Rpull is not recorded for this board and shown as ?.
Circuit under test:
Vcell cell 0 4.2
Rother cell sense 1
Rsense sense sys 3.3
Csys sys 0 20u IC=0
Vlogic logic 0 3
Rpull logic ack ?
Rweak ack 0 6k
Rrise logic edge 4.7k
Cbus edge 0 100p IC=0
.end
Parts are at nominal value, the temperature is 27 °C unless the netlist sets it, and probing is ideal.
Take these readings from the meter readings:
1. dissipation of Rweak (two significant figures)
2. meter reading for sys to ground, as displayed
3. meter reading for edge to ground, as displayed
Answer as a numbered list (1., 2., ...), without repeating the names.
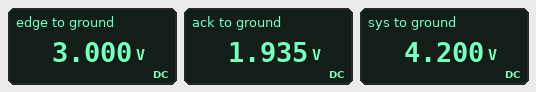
1. 620 µW
2. 4.200 V
3. 3.000 V
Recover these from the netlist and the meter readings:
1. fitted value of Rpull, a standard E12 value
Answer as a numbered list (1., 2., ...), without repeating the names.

1. 3.3 kΩ
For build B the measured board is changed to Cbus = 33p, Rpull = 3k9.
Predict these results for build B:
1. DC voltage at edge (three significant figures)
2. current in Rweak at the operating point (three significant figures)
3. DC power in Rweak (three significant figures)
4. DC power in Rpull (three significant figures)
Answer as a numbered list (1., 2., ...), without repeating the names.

1. 3.00 V
2. 303 µA
3. 551 µW
4. 358 µW
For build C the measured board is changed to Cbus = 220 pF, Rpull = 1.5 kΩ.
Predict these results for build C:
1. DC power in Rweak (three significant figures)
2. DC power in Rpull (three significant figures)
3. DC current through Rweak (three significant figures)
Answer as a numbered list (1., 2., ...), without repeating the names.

1. 960 µW
2. 240 µW
3. 400 µA
